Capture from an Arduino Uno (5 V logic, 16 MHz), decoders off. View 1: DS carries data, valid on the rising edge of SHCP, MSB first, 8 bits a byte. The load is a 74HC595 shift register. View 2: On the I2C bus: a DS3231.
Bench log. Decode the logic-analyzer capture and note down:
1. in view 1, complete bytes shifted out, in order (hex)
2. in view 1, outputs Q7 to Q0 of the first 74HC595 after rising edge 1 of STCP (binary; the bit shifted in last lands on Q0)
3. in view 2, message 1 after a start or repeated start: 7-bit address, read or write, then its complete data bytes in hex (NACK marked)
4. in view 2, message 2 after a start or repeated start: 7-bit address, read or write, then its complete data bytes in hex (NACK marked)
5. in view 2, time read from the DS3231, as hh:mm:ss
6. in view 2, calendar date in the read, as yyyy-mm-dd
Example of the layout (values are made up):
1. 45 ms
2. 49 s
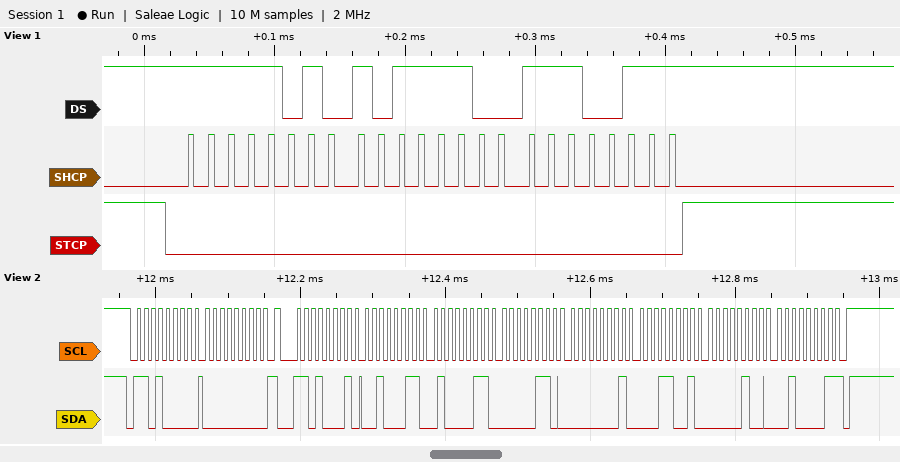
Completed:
1. FA BC E7
2. 11100111
3. 0x68 write: 00
4. 0x68 read: 23 43 06 01 19 04 21 NACK
5. 06:43:23
6. 2021-04-19
